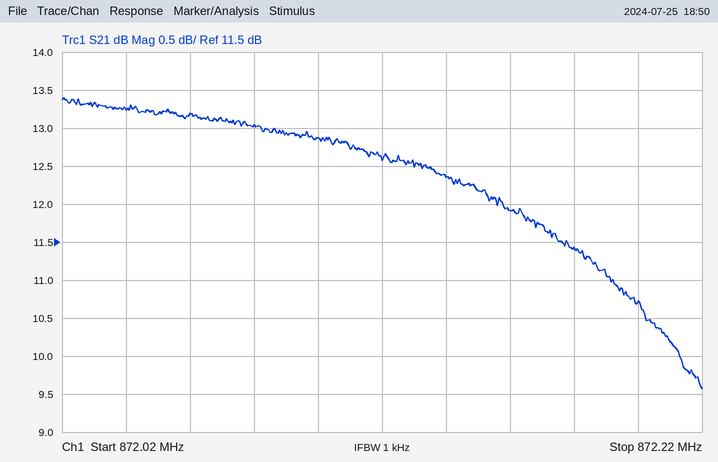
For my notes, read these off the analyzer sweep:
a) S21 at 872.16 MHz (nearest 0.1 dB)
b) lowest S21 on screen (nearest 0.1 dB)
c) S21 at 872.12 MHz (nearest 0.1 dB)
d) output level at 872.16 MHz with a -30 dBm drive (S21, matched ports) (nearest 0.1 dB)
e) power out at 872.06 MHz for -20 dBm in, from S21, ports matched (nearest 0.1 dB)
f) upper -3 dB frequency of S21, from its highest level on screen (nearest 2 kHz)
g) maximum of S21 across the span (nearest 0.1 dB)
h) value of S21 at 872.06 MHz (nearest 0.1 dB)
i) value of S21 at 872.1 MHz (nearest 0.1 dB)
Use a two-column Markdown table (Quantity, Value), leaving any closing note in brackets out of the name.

| Quantity | Value |
|---|---|
| S21 at 872.16 MHz | 11.9 dB |
| lowest S21 on screen | 9.6 dB |
| S21 at 872.12 MHz | 12.6 dB |
| output level at 872.16 MHz with a -30 dBm drive (S21, matched ports) | -18.1 dBm |
| power out at 872.06 MHz for -20 dBm in, from S21, ports matched | -6.8 dBm |
| upper -3 dB frequency of S21, from its highest level on screen | 872.206 MHz |
| maximum of S21 across the span | 13.4 dB |
| value of S21 at 872.06 MHz | 13.2 dB |
| value of S21 at 872.1 MHz | 12.9 dB |
